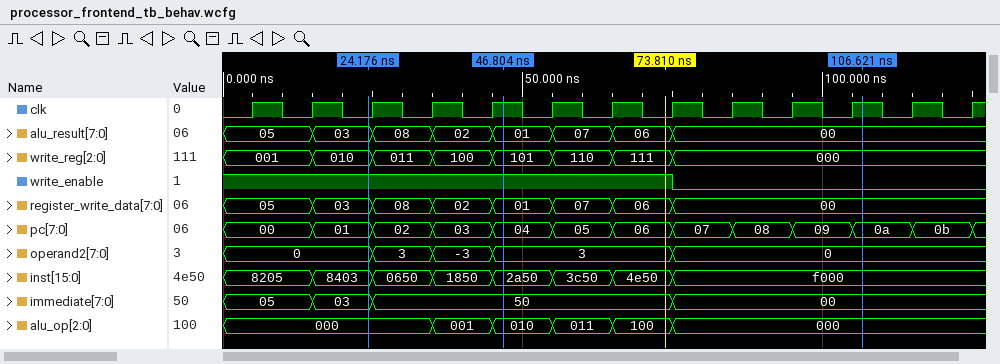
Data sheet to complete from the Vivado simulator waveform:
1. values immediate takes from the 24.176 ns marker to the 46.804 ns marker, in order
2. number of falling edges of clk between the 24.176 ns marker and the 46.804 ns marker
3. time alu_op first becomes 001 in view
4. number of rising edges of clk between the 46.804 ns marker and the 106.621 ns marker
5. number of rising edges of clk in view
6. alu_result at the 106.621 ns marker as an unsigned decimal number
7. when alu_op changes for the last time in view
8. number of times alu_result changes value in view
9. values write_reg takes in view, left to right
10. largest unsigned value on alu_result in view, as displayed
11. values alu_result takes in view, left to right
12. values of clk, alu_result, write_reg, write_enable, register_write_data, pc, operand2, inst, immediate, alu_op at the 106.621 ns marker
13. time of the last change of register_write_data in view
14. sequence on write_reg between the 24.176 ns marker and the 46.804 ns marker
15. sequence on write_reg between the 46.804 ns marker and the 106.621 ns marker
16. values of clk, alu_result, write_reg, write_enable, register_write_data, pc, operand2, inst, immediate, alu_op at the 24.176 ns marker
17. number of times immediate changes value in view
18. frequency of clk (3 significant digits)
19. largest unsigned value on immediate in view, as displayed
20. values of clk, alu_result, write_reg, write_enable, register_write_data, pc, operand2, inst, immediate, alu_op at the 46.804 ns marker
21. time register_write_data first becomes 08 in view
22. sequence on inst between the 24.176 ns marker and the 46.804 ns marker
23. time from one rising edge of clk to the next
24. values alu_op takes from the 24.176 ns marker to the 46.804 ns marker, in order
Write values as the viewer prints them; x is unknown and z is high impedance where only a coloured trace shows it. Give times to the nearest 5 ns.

03, 50
2
35 ns
6
13
0
75 ns
7
001, 010, 011, 100, 101, 110, 111, 000
08
05, 03, 08, 02, 01, 07, 06, 00
clk=1, alu_result=00, write_reg=000, write_enable=0, register_write_data=00, pc=0a, operand2=0, inst=f000, immediate=00, alu_op=000
75 ns
010, 011, 100, 101
101, 110, 111, 000
clk=0, alu_result=03, write_reg=010, write_enable=1, register_write_data=03, pc=01, operand2=0, inst=8403, immediate=03, alu_op=000
3
100 MHz
50
clk=1, alu_result=01, write_reg=101, write_enable=1, register_write_data=01, pc=04, operand2=3, inst=2a50, immediate=50, alu_op=010
25 ns
8403, 0650, 1850, 2a50
10 ns
000, 001, 010
